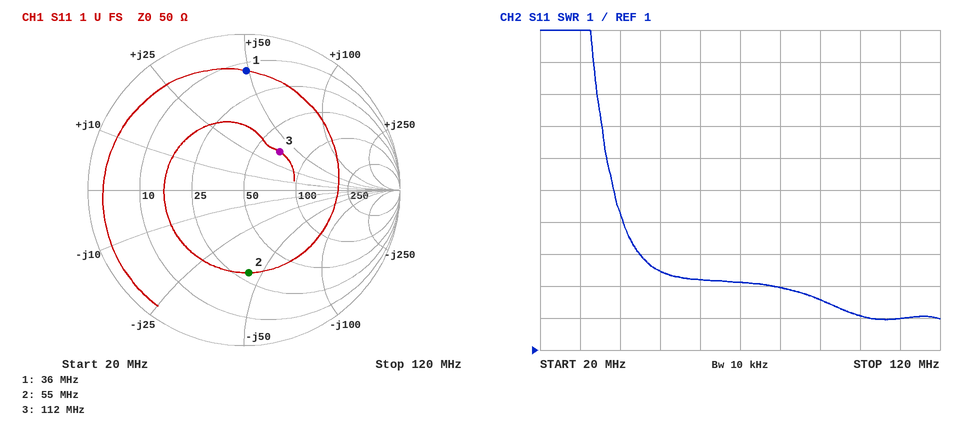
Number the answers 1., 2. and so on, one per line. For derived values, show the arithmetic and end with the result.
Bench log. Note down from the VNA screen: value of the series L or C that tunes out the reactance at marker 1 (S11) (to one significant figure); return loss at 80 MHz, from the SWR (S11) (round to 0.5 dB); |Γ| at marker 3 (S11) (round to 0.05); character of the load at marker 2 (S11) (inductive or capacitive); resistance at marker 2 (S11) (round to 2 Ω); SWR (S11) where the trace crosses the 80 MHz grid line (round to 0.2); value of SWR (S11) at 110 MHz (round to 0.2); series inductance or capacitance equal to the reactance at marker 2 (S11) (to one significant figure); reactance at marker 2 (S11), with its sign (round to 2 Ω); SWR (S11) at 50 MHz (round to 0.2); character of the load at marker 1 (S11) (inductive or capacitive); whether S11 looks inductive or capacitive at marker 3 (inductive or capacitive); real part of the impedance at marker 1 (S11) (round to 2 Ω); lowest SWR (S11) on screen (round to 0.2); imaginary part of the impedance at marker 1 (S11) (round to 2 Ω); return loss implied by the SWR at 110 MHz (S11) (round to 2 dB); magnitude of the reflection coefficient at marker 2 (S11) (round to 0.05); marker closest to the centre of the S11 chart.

1. C = 1/(2π × 36 MHz × 50 Ω) ≈ 88.4 pF, so 90 pF to one significant figure
2. −20 log10((3 − 1)/(3 + 1)) ≈ 6.0 dB
3. 0.35
4. capacitive
5. 30 Ω
6. 3.0
7. 2.0
8. C = 1/(2π × 55 MHz × 44 Ω) ≈ 65.8 pF, so 70 pF to one significant figure
9. -44 Ω
10. 3.4
11. inductive
12. inductive
13. 14 Ω
14. 2.0
15. +50 Ω
16. −20 log10((2 − 1)/(2 + 1)) ≈ 10 dB
17. 0.55
18. marker 3
